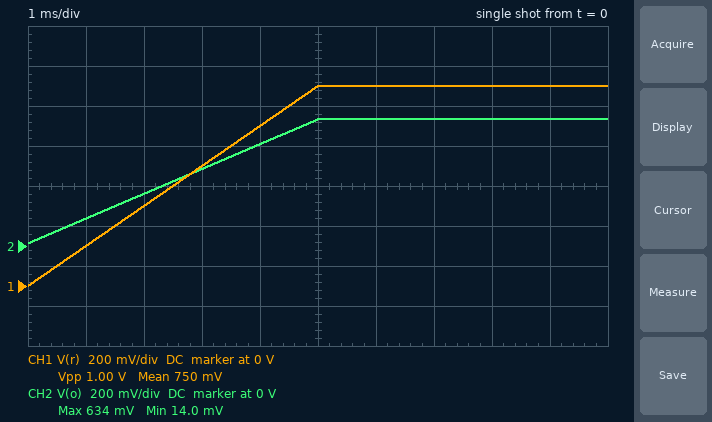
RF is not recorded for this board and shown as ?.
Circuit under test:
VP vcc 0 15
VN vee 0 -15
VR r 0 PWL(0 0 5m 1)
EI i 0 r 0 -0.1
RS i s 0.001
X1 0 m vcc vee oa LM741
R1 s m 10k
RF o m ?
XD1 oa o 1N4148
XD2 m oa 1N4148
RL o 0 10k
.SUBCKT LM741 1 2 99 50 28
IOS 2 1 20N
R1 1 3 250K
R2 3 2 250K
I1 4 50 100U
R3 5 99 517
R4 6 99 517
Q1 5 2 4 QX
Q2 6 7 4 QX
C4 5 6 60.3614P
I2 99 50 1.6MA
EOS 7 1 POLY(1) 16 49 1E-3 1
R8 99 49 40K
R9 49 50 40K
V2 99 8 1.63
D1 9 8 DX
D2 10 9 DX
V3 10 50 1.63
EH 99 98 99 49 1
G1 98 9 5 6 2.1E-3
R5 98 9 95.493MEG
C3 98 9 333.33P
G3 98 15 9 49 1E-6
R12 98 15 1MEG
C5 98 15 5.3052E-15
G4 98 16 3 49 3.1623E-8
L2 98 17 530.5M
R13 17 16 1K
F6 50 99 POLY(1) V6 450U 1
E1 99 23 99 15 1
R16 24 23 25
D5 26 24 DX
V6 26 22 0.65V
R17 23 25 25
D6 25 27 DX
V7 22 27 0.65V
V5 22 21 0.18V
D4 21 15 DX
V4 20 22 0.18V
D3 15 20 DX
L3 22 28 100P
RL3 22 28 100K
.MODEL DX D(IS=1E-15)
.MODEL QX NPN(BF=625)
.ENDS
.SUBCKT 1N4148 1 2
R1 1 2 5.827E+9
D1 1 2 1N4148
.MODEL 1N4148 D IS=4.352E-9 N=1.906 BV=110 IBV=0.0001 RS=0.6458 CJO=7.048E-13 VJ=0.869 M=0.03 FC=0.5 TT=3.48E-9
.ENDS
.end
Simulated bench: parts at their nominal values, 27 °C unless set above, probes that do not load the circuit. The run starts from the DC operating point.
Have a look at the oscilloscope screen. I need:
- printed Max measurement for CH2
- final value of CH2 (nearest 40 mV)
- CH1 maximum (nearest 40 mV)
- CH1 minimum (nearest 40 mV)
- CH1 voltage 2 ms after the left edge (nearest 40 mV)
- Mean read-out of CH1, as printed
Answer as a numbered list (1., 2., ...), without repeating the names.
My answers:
1. 634 mV
2. 640 mV
3. 1.00 V
4. 0 V
5. 400 mV
6. 750 mV
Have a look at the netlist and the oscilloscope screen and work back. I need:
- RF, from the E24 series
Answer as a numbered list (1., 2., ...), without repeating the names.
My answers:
1. 62 kΩ
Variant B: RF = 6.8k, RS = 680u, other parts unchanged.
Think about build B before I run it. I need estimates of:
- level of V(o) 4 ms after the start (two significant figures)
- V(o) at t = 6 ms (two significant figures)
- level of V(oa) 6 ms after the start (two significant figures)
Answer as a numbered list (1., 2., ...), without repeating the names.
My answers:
1. 57 mV
2. 70 mV
3. 480 mV
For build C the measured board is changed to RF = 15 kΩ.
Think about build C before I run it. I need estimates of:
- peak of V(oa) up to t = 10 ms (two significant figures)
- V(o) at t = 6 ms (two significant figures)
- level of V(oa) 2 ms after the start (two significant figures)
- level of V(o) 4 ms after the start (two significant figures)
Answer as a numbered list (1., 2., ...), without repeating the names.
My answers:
1. 580 mV
2. 150 mV
3. 450 mV
4. 120 mV
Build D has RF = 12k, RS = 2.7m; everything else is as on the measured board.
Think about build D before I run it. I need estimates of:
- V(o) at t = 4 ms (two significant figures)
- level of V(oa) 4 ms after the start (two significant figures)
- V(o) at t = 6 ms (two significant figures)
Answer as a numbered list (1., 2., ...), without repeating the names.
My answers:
1. 99 mV
2. 510 mV
3. 120 mV
